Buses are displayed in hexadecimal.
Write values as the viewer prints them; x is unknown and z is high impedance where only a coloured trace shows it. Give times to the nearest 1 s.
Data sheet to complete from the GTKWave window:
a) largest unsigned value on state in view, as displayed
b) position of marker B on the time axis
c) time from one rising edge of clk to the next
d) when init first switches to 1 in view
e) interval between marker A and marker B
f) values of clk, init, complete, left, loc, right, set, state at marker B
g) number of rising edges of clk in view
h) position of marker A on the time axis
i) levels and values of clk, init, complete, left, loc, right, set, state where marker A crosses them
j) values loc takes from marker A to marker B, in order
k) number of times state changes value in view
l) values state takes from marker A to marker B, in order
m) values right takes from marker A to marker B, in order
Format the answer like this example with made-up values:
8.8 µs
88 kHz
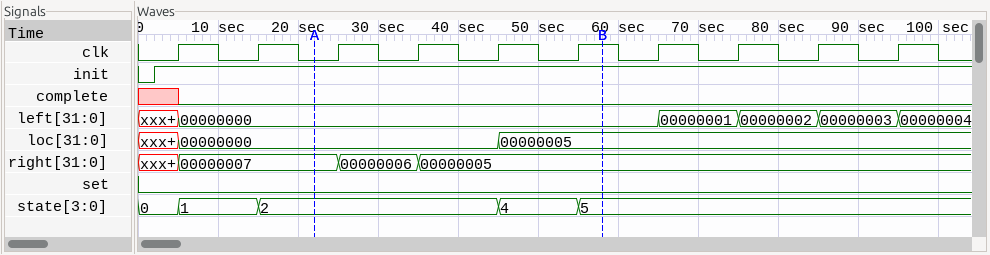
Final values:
5
58 s
10 s
2 s
36 s
clk=1, init=1, complete=0, left=00000000, loc=00000005, right=00000005, set=0, state=5
10
22 s
clk=0, init=1, complete=0, left=00000000, loc=00000000, right=00000007, set=0, state=2
00000000, 00000005
4
2, 4, 5
00000007, 00000006, 00000005
